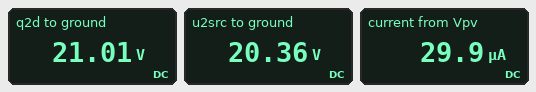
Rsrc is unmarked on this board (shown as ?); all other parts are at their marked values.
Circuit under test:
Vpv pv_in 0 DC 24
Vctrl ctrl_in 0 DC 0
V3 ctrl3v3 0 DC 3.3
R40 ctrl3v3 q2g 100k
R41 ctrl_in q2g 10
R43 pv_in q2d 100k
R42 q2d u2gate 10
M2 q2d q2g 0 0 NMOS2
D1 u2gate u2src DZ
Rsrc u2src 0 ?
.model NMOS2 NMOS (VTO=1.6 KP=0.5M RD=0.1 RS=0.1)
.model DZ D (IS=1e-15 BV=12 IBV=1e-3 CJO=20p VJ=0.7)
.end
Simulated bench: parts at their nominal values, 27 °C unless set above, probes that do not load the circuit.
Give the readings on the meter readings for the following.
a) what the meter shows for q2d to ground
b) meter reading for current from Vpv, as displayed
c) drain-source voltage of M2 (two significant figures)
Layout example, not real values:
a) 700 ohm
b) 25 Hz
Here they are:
a) 21.01 V
b) 29.9 µA
c) 21 V
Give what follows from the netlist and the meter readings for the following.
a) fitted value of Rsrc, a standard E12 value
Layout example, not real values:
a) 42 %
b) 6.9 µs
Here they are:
a) 680 kΩ
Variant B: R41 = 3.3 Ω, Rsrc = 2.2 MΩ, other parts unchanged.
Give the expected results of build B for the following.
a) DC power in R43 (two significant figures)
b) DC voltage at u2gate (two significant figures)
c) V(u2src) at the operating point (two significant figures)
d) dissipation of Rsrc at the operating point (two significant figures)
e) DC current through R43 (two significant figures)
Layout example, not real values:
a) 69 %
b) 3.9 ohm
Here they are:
a) 10 µW
b) 23 V
c) 22 V
d) 230 µW
e) 10 µA
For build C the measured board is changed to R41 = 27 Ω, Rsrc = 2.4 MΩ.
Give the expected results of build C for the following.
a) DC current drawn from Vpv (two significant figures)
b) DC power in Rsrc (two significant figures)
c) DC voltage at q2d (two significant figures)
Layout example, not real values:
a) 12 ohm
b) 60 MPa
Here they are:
a) 9.4 µA
b) 210 µW
c) 23 V
